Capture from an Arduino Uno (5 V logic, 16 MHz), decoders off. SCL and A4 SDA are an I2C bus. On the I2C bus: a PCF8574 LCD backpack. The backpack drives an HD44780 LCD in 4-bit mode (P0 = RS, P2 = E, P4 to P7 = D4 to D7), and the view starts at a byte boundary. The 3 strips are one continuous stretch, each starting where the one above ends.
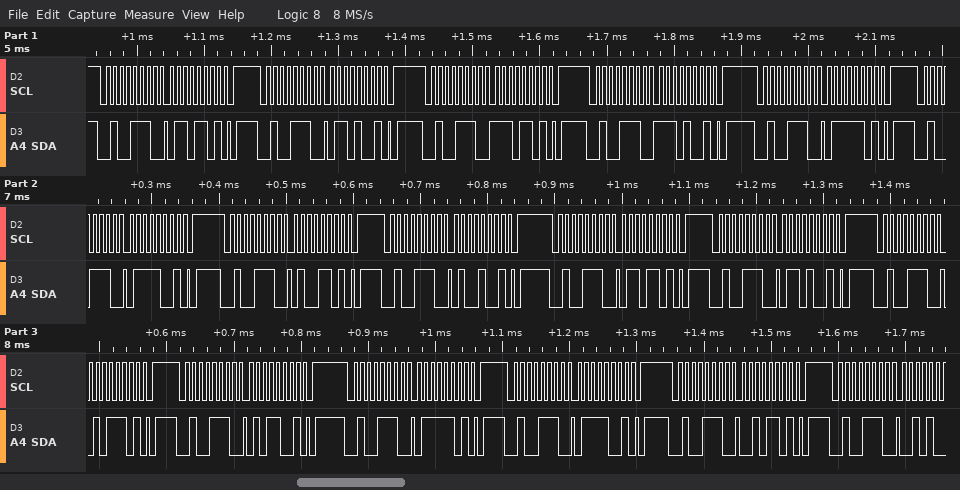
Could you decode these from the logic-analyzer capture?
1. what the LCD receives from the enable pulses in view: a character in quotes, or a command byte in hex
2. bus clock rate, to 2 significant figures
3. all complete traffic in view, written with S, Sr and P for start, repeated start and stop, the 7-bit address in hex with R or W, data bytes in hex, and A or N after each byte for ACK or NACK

'n' 't' 'e'
100 kHz
S 27W A 6D A P S 27W A 69 A P S 27W A ED A P S 27W A E9 A P S 27W A 7D A P S 27W A 79 A P S 27W A 4D A P S 27W A 49 A P S 27W A 6D A P S 27W A 69 A P S 27W A 5D A P S 27W A 59 A P S 27W A 7D A P S 27W A 79 A P S 27W A 2D A P S 27W A
